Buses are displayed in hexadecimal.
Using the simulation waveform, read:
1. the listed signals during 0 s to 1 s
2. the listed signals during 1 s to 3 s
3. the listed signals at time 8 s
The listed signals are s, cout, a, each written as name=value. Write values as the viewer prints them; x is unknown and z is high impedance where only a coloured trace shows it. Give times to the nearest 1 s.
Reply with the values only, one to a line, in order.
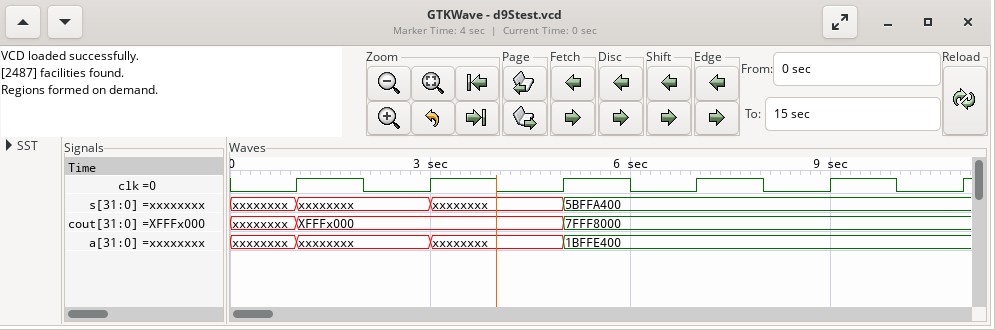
s=xxxxxxxx, cout=xxxxxxxx, a=xxxxxxxx
s=xxxxxxxx, cout=XFFFx000, a=xxxxxxxx
s=5BFFA400, cout=7FFF8000, a=1BFFE400
